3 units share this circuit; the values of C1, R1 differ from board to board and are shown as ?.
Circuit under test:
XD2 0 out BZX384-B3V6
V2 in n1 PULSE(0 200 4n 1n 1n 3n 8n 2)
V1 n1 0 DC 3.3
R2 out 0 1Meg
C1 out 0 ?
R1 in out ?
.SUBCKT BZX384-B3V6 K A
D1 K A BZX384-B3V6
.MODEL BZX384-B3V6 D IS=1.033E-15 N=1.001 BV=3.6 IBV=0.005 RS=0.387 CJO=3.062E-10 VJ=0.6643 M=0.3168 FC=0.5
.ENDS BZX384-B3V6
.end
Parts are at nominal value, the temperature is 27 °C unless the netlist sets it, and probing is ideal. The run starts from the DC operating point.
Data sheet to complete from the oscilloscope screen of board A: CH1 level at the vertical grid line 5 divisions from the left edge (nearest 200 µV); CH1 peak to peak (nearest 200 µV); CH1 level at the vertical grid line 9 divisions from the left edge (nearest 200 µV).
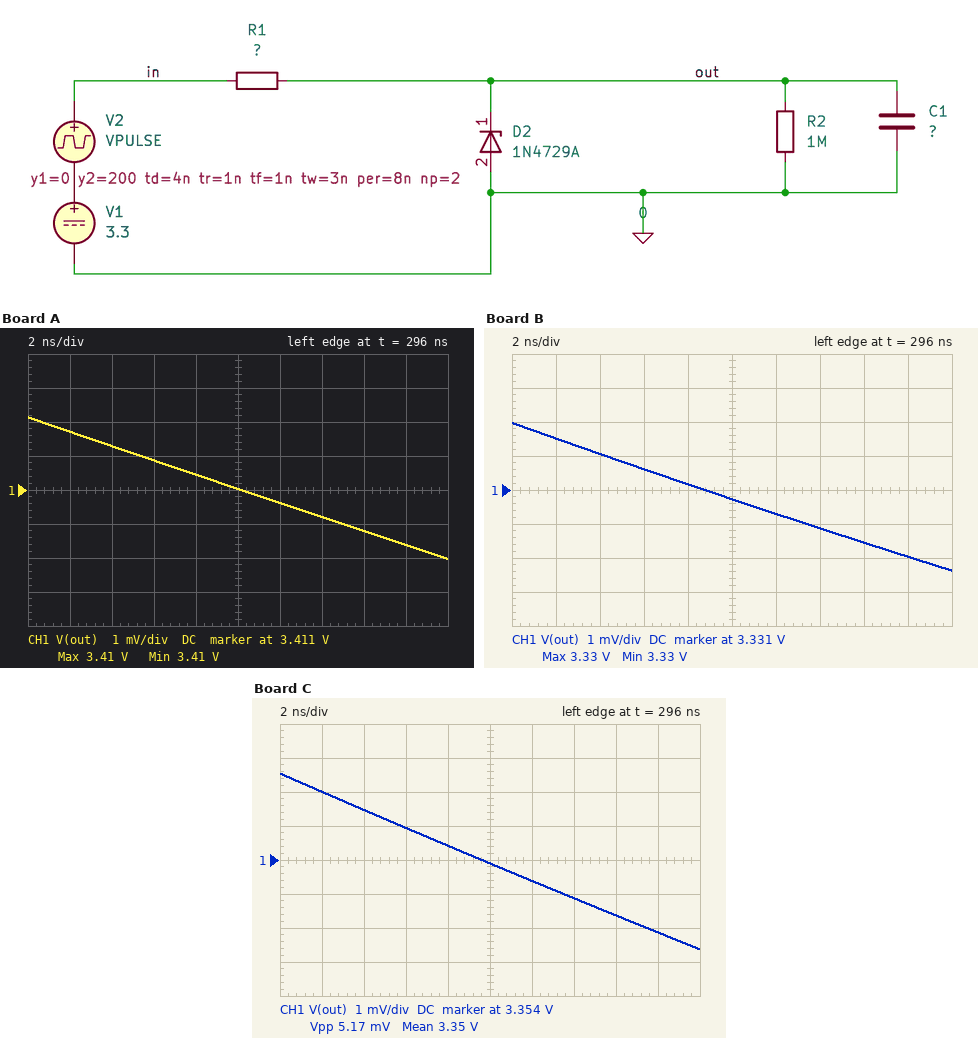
3.4110 V
4.2 mV
3.4094 V
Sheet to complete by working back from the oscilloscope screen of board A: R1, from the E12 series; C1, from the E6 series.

3.3 kΩ
22 pF
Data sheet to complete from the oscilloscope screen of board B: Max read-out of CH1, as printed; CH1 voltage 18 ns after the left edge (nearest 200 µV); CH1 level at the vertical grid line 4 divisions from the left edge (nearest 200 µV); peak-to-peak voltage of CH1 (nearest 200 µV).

3.33 V
3.3290 V
3.3312 V
4.4 mV
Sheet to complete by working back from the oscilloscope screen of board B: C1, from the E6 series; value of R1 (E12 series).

15 pF
820 Ω
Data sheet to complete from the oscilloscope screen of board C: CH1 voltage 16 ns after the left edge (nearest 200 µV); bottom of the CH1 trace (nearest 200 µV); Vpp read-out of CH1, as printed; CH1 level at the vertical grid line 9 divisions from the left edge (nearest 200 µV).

3.3524 V
3.3514 V
5.17 mV
3.3518 V
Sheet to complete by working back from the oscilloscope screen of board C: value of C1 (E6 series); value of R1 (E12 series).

15 pF
1.2 kΩ
